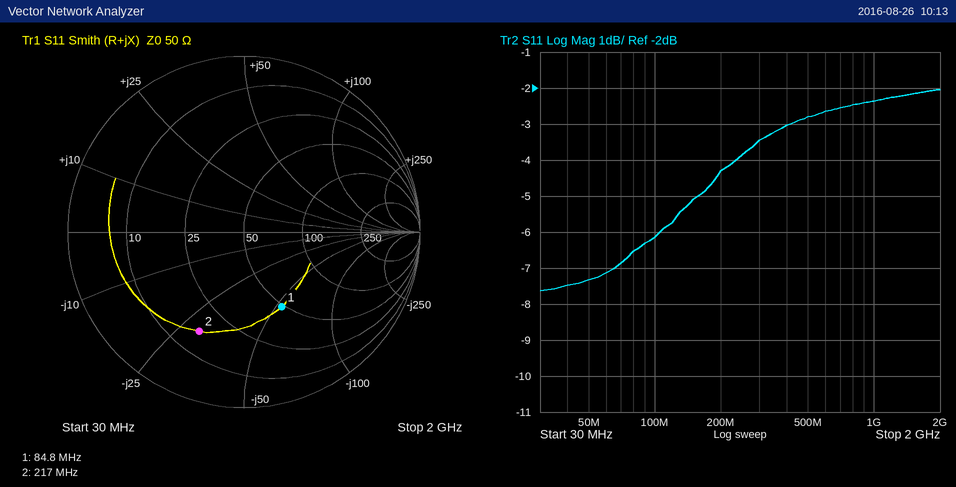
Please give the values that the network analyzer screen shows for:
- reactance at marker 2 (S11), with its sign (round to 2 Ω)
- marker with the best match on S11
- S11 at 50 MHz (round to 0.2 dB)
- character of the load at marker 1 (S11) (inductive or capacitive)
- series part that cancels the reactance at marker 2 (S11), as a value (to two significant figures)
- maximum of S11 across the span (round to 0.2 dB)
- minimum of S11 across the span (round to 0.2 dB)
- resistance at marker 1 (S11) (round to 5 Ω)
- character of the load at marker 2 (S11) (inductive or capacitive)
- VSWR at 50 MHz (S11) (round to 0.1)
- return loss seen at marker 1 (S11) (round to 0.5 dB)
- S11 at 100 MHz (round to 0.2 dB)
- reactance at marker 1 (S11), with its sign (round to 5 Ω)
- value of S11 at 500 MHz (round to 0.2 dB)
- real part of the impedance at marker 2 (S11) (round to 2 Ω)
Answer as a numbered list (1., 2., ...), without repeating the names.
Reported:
1. -30 Ω
2. marker 1
3. -7.4 dB
4. capacitive
5. 22 nH
6. -2.0 dB
7. -7.6 dB
8. 50 Ω
9. capacitive
10. 2.5
11. 6.5 dB
12. -6.2 dB
13. -55 Ω
14. -2.8 dB
15. 16 Ω
